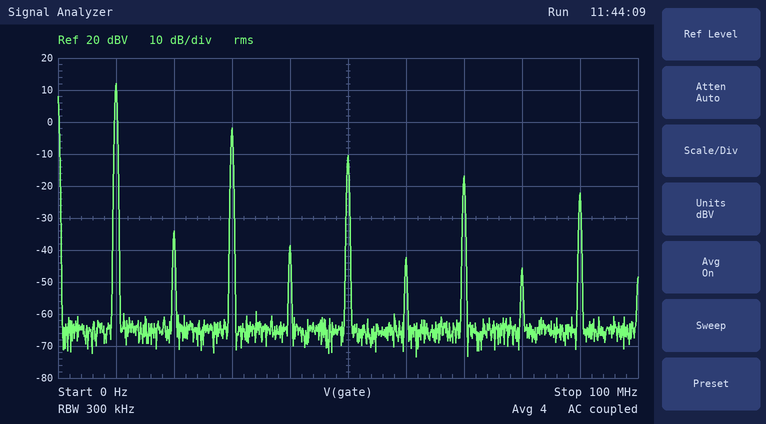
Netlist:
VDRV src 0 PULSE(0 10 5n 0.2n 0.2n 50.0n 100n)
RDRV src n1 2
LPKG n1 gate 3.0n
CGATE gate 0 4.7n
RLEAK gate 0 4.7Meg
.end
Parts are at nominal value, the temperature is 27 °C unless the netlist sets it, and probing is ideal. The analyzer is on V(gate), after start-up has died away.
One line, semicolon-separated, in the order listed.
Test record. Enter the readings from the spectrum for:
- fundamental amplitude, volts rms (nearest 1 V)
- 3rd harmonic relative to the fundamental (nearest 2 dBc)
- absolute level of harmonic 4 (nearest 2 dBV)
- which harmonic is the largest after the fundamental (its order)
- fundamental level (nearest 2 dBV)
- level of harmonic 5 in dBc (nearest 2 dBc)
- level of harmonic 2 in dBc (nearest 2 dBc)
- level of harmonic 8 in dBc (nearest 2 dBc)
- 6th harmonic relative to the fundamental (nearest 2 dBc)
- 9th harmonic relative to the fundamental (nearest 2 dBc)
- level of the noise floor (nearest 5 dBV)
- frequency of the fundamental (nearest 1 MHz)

4 V; -14 dBc; -38 dBV; 3; 12 dBV; -22 dBc; -46 dBc; -58 dBc; -54 dBc; -34 dBc; -65 dBV; 10 MHz
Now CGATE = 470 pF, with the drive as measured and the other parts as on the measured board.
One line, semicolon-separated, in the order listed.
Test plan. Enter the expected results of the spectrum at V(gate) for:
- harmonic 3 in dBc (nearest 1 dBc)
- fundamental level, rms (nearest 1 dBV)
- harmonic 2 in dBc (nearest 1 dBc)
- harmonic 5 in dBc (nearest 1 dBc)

-9 dBc; 13 dBV; -44 dBc; -13 dBc
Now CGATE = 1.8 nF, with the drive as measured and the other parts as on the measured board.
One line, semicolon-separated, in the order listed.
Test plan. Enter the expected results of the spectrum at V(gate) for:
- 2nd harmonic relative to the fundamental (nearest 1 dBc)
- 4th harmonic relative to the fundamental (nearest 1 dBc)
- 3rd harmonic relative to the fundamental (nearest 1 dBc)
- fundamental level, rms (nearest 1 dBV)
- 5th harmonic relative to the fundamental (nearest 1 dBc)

-44 dBc; -45 dBc; -10 dBc; 13 dBV; -16 dBc
